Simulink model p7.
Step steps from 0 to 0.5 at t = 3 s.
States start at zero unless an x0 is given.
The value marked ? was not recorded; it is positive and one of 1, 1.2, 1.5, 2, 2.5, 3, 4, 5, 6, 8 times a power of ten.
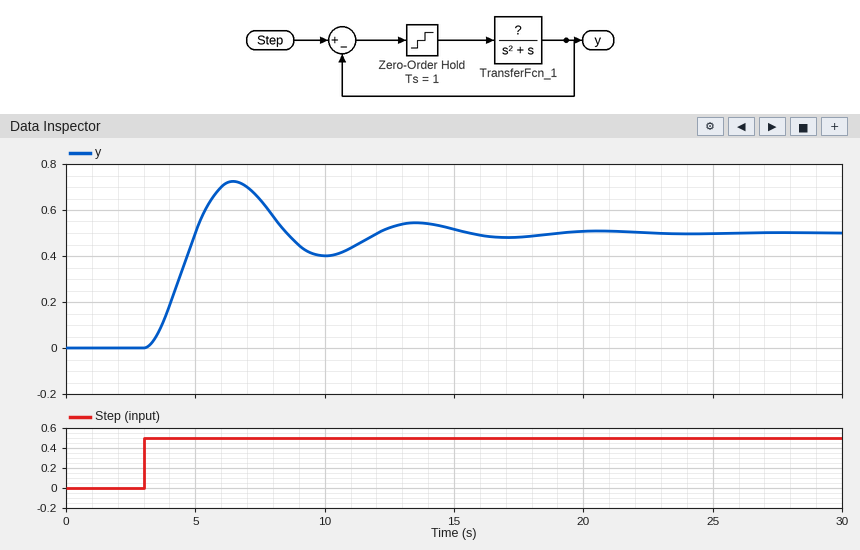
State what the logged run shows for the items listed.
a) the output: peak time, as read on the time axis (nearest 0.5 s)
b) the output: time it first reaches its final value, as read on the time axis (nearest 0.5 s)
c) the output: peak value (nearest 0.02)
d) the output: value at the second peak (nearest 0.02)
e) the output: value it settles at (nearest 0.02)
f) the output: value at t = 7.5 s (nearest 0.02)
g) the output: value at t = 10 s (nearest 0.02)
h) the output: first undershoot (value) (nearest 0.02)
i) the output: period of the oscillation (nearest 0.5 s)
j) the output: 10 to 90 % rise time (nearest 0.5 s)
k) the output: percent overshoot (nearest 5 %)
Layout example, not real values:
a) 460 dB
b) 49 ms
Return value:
a) 6.5 s
b) 5.0 s
c) 0.72
d) 0.54
e) 0.50
f) 0.64
g) 0.40
h) 0.40
i) 7.0 s
j) 1.5 s
k) 45 %
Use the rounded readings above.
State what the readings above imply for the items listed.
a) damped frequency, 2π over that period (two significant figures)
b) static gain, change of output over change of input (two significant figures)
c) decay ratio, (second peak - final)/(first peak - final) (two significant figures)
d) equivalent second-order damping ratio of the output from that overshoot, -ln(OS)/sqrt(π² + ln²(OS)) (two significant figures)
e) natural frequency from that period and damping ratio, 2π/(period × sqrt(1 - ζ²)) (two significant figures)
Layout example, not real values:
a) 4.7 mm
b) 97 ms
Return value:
a) 0.90 rad/s
b) 1.0
c) 0.18
d) 0.25
e) 0.93 rad/s
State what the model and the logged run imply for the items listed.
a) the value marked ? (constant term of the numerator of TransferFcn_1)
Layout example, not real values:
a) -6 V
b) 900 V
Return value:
a) 1
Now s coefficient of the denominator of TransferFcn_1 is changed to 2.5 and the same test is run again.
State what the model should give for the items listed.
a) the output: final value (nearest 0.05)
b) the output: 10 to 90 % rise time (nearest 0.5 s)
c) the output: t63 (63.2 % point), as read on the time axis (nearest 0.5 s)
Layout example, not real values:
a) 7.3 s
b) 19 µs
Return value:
a) 0.50
b) 3.5 s
c) 5.0 s
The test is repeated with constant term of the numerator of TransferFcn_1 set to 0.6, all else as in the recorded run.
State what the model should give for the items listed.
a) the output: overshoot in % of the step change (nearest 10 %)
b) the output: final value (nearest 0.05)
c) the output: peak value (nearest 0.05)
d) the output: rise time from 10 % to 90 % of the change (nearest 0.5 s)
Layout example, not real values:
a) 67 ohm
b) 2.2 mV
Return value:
a) 20 %
b) 0.50
c) 0.60
d) 2.0 s
